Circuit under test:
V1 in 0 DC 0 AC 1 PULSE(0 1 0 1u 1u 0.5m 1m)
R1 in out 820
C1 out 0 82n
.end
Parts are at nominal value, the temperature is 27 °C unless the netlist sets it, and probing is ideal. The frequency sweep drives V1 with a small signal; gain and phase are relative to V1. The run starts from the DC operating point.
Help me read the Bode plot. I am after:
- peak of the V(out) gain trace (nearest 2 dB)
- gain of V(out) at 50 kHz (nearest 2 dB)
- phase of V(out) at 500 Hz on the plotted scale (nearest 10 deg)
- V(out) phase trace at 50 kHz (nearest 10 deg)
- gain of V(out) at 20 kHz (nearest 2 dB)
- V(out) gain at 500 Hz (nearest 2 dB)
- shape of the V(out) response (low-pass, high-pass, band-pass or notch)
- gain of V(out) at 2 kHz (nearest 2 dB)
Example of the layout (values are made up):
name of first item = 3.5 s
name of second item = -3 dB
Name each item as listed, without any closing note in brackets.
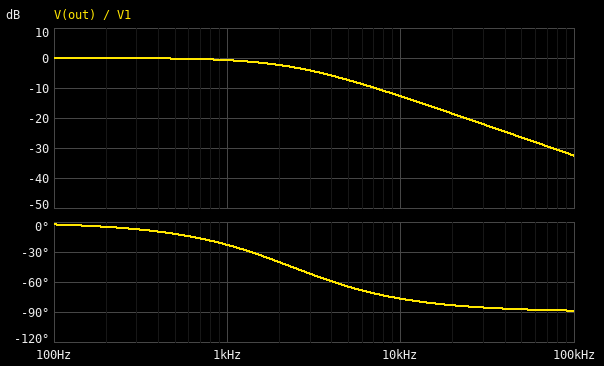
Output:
peak of the V(out) gain trace = 0 dB
gain of V(out) at 50 kHz = -26 dB
phase of V(out) at 500 Hz on the plotted scale = -10 deg
V(out) phase trace at 50 kHz = -90 deg
gain of V(out) at 20 kHz = -18 dB
V(out) gain at 500 Hz = 0 dB
shape of the V(out) response = low-pass
gain of V(out) at 2 kHz = -2 dB
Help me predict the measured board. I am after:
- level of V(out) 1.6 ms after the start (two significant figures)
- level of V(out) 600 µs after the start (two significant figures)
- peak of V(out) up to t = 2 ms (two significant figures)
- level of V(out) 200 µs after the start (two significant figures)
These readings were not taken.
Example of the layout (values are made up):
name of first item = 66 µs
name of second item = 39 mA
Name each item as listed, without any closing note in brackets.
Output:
level of V(out) 1.6 ms after the start = 230 mV
level of V(out) 600 µs after the start = 230 mV
peak of V(out) up to t = 2 ms = 1.0 V
level of V(out) 200 µs after the start = 950 mV
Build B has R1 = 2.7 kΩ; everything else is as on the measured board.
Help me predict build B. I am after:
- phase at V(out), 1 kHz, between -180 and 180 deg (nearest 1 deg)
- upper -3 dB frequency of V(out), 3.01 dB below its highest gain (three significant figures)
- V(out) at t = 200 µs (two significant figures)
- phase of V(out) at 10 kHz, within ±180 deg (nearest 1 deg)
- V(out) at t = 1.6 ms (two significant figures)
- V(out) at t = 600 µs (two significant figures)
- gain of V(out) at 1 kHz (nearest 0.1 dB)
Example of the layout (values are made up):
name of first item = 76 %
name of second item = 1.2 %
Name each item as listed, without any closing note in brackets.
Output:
phase at V(out), 1 kHz, between -180 and 180 deg = -54 deg
upper -3 dB frequency of V(out), 3.01 dB below its highest gain = 719 Hz
V(out) at t = 200 µs = 590 mV
phase of V(out) at 10 kHz, within ±180 deg = -86 deg
V(out) at t = 1.6 ms = 580 mV
V(out) at t = 600 µs = 570 mV
gain of V(out) at 1 kHz = -4.7 dB
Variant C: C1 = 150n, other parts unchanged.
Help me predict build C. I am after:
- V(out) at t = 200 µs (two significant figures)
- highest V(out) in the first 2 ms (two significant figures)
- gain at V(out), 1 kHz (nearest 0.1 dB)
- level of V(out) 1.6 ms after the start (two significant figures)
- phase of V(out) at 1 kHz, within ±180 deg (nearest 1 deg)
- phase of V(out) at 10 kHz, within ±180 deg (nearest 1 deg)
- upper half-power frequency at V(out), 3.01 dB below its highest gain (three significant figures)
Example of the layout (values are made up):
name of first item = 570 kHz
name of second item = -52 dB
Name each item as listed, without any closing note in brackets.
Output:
V(out) at t = 200 µs = 800 mV
highest V(out) in the first 2 ms = 980 mV
gain at V(out), 1 kHz = -2.0 dB
level of V(out) 1.6 ms after the start = 440 mV
phase of V(out) at 1 kHz, within ±180 deg = -38 deg
phase of V(out) at 10 kHz, within ±180 deg = -83 deg
upper half-power frequency at V(out), 3.01 dB below its highest gain = 1.29 kHz
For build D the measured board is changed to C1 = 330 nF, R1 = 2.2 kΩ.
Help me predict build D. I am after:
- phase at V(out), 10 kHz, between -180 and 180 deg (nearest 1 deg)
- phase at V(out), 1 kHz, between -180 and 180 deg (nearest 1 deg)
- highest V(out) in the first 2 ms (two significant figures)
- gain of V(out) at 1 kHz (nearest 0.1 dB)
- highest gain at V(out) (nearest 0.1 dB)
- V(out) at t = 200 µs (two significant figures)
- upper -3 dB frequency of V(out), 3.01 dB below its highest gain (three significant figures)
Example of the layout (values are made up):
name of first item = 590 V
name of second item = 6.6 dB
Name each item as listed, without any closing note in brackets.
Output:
phase at V(out), 10 kHz, between -180 and 180 deg = -89 deg
phase at V(out), 1 kHz, between -180 and 180 deg = -78 deg
highest V(out) in the first 2 ms = 620 mV
gain of V(out) at 1 kHz = -13.4 dB
highest gain at V(out) = 0 dB
V(out) at t = 200 µs = 240 mV
upper -3 dB frequency of V(out), 3.01 dB below its highest gain = 219 Hz
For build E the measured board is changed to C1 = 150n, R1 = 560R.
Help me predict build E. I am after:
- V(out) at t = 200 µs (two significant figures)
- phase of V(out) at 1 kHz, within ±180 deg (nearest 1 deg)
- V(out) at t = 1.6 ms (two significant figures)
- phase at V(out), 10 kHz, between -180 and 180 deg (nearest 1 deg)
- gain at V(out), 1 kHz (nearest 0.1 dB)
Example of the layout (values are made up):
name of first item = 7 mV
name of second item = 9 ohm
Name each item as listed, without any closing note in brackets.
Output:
V(out) at t = 200 µs = 910 mV
phase of V(out) at 1 kHz, within ±180 deg = -28 deg
V(out) at t = 1.6 ms = 310 mV
phase at V(out), 10 kHz, between -180 and 180 deg = -79 deg
gain at V(out), 1 kHz = -1.1 dB
